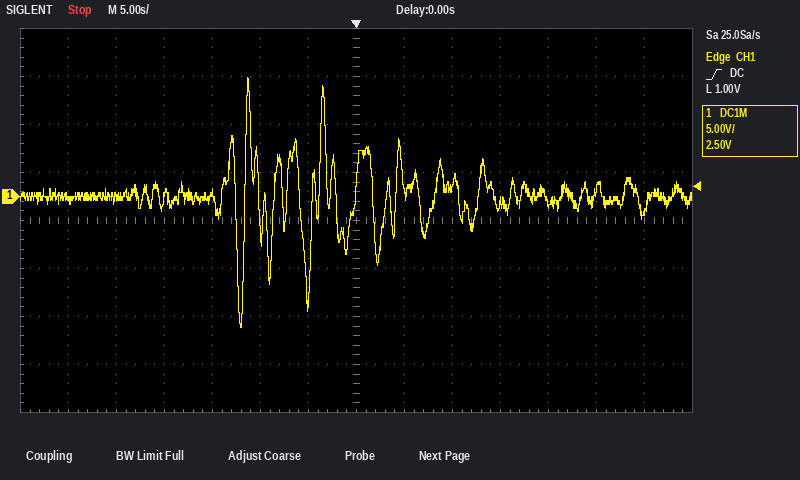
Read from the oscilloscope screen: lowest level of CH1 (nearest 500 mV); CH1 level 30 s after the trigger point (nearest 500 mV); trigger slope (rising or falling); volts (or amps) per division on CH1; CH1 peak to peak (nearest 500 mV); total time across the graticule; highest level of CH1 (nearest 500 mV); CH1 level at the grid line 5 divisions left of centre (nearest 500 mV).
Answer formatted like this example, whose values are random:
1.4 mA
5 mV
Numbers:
-13.5 V
-1.5 V
rising
5 V
26.0 V
70 s
12.5 V
0.0 V
